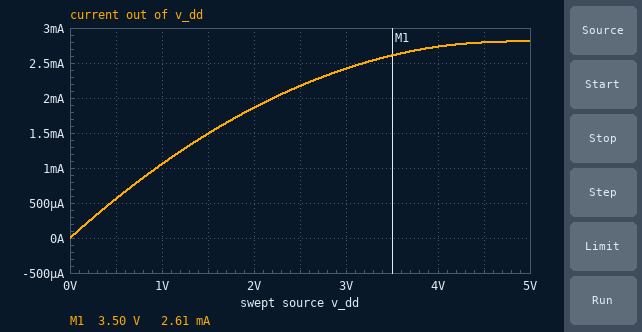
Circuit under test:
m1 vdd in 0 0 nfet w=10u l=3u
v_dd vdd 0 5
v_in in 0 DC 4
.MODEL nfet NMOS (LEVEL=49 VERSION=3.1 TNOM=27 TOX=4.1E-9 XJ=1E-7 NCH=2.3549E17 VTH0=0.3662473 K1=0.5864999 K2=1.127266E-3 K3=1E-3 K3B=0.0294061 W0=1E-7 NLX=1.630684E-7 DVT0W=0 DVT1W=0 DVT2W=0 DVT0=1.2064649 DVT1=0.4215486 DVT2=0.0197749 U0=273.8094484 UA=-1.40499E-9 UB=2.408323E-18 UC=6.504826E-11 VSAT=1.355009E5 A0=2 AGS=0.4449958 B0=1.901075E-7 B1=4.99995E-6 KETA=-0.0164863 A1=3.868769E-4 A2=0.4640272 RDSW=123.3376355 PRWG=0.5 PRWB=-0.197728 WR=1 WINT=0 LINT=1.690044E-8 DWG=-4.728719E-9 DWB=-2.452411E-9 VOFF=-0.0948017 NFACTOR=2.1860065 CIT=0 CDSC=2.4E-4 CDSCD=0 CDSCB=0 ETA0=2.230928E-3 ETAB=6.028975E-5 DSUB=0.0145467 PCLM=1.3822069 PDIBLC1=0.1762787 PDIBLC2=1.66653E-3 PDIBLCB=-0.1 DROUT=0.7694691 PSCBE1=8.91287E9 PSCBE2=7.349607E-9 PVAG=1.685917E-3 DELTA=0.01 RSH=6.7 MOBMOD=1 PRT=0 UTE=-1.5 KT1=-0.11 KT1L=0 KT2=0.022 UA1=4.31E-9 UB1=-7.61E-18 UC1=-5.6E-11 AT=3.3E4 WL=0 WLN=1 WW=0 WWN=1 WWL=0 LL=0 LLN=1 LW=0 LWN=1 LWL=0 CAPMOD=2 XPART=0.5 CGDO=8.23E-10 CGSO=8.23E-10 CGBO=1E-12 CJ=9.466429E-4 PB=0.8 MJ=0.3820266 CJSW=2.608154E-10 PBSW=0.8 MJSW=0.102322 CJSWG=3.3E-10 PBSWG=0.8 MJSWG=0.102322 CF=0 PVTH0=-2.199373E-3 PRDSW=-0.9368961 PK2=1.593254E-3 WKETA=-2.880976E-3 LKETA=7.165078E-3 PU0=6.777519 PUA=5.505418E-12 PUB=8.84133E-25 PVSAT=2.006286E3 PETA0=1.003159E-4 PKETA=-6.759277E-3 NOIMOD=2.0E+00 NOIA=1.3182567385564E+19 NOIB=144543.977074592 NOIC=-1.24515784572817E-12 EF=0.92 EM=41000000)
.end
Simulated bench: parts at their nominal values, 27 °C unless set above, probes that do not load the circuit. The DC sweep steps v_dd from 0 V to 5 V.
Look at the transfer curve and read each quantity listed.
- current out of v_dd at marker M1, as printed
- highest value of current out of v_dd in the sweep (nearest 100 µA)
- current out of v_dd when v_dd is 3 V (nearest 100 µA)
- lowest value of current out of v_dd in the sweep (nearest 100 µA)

2.61 mA
2.8 mA
2.4 mA
0 A
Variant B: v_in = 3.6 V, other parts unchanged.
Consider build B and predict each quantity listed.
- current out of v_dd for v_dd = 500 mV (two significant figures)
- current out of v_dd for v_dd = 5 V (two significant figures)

580 µA
2.4 mA
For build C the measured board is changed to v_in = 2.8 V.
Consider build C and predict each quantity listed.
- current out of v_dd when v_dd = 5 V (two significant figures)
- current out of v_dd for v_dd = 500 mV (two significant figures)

1.6 mA
580 µA
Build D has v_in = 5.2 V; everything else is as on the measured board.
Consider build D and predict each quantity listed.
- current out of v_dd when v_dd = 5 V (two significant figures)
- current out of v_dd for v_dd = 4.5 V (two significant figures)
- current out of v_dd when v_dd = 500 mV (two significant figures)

3.7 mA
3.5 mA
490 µA
